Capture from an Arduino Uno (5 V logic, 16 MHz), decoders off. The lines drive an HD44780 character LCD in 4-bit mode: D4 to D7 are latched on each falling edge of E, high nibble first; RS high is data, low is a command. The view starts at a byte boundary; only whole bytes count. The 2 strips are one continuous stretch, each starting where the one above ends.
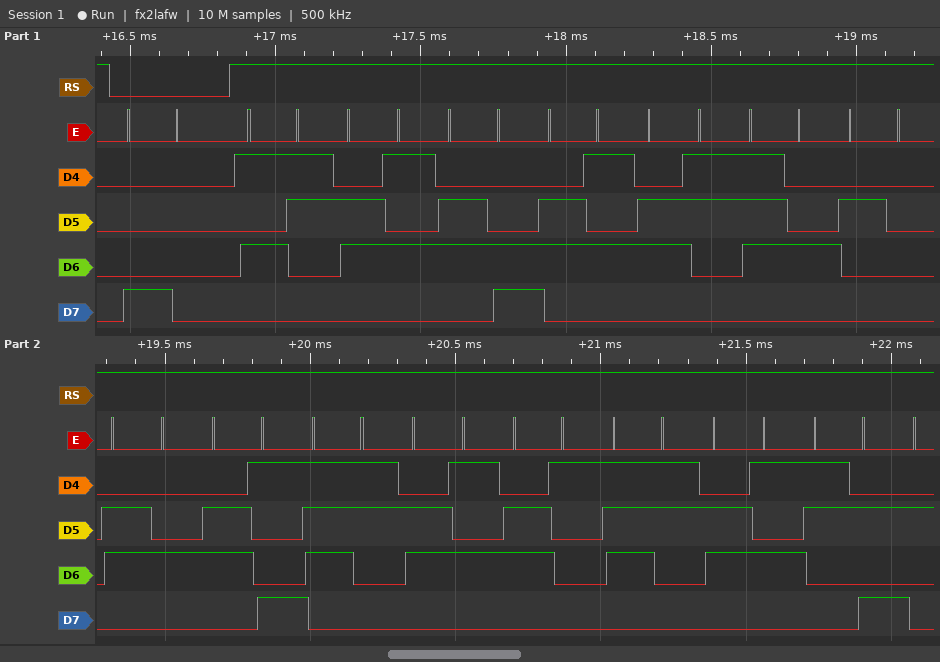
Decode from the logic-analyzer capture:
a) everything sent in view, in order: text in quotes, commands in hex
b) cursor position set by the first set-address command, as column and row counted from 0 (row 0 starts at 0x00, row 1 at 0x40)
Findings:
0x80 "Select disease:"
column 0, row 0
